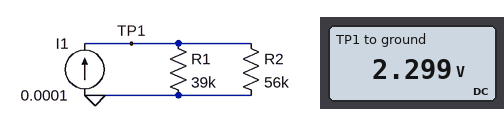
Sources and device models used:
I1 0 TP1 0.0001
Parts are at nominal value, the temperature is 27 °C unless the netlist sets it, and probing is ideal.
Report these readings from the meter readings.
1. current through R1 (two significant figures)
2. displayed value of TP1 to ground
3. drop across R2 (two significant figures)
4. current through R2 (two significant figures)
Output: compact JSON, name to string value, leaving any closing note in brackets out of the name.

{"current through R1": "59 µA", "displayed value of TP1 to ground": "2.299 V", "drop across R2": "2.3 V", "current through R2": "41 µA"}
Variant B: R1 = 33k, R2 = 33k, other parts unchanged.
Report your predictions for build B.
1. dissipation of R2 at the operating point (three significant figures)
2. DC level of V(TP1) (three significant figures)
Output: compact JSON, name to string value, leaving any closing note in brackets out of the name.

{"dissipation of R2 at the operating point": "82.5 µW", "DC level of V(TP1)": "1.65 V"}
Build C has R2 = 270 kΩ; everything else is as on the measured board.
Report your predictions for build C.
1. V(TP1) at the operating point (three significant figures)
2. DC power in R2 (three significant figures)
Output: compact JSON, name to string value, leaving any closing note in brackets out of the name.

{"V(TP1) at the operating point": "3.41 V", "DC power in R2": "43.0 µW"}
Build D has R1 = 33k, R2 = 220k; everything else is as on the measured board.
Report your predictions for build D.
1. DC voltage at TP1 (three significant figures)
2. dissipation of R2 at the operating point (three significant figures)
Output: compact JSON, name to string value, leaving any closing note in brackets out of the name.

{"DC voltage at TP1": "2.87 V", "dissipation of R2 at the operating point": "37.4 µW"}
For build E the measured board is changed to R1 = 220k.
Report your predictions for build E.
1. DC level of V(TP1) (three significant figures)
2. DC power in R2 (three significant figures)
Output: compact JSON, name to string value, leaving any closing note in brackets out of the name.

{"DC level of V(TP1)": "4.46 V", "DC power in R2": "356 µW"}
